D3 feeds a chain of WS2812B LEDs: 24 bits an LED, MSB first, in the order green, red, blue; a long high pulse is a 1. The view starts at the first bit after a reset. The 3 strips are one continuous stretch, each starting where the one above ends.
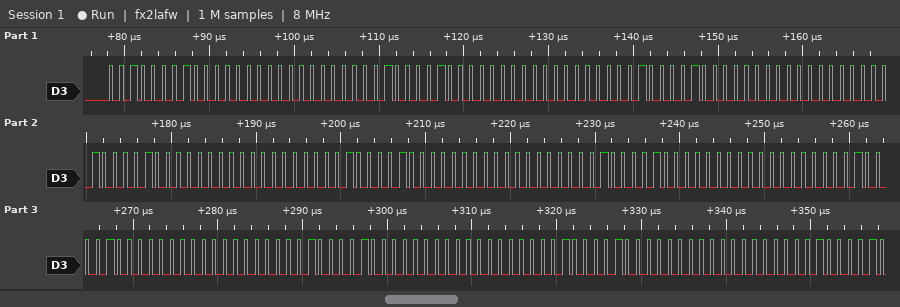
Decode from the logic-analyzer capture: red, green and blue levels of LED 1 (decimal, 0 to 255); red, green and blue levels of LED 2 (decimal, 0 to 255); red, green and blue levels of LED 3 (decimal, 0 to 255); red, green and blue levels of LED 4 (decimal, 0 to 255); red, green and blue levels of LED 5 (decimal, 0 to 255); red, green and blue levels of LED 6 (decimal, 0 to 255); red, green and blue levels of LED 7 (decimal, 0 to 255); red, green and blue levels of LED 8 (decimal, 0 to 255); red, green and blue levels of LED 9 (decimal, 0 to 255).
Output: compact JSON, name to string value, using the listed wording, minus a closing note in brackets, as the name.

{"red, green and blue levels of LED 1": "0, 33, 0", "red, green and blue levels of LED 2": "0, 33, 0", "red, green and blue levels of LED 3": "0, 33, 0", "red, green and blue levels of LED 4": "0, 33, 0", "red, green and blue levels of LED 5": "0, 33, 0", "red, green and blue levels of LED 6": "0, 33, 0", "red, green and blue levels of LED 7": "0, 33, 0", "red, green and blue levels of LED 8": "0, 33, 0", "red, green and blue levels of LED 9": "0, 33, 0"}
